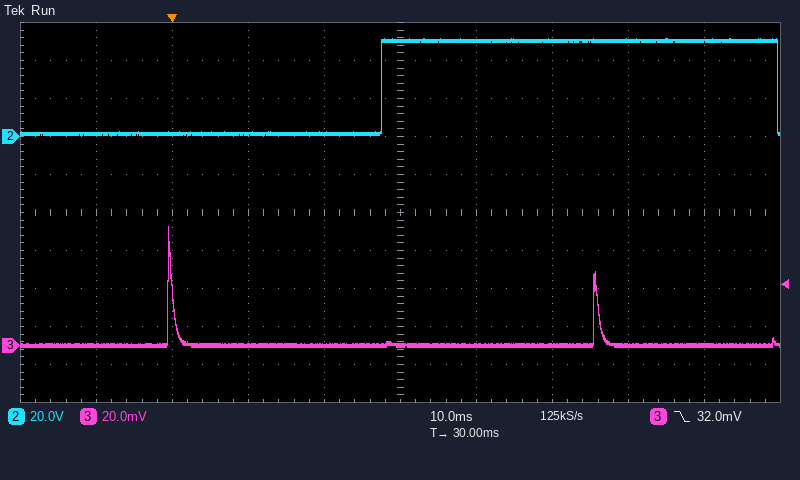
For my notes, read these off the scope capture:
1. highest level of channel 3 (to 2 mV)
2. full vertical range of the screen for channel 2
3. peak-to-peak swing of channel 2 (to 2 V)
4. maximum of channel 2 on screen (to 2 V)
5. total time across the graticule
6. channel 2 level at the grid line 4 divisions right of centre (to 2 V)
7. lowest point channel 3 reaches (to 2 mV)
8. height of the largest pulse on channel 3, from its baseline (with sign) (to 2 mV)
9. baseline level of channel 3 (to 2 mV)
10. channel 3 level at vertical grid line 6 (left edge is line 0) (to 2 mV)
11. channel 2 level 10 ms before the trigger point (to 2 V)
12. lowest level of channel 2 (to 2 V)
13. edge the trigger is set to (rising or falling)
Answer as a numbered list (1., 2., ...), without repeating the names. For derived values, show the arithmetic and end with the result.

1. 62 mV
2. 200 V
3. 52 V − (2 V) = 50 V
4. 52 V
5. 100 ms
6. 50 V
7. 0 mV
8. 62 mV − (0 mV) = +62 mV
9. 0 mV
10. 0 mV
11. 2 V
12. 2 V
13. falling
